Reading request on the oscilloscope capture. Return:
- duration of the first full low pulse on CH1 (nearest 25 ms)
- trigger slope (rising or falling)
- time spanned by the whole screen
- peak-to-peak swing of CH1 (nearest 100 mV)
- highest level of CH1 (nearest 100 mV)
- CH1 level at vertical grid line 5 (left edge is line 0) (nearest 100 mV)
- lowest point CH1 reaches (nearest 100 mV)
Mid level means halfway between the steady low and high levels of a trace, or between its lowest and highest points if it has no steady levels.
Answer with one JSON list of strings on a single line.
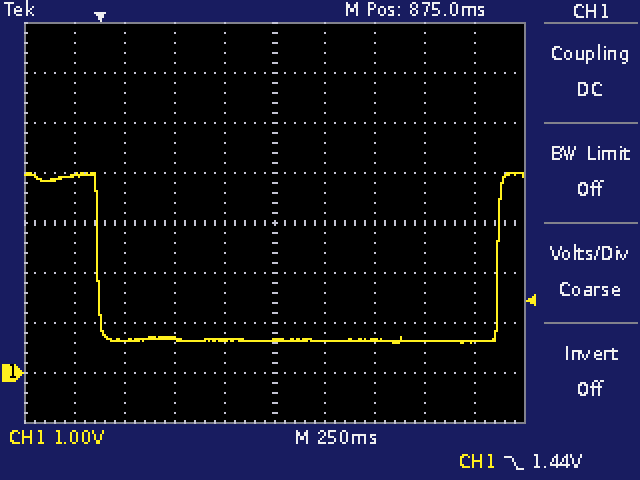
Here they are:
["2.000 s", "falling", "2.5 s", "3.4 V", "4.0 V", "700 mV", "600 mV"]
